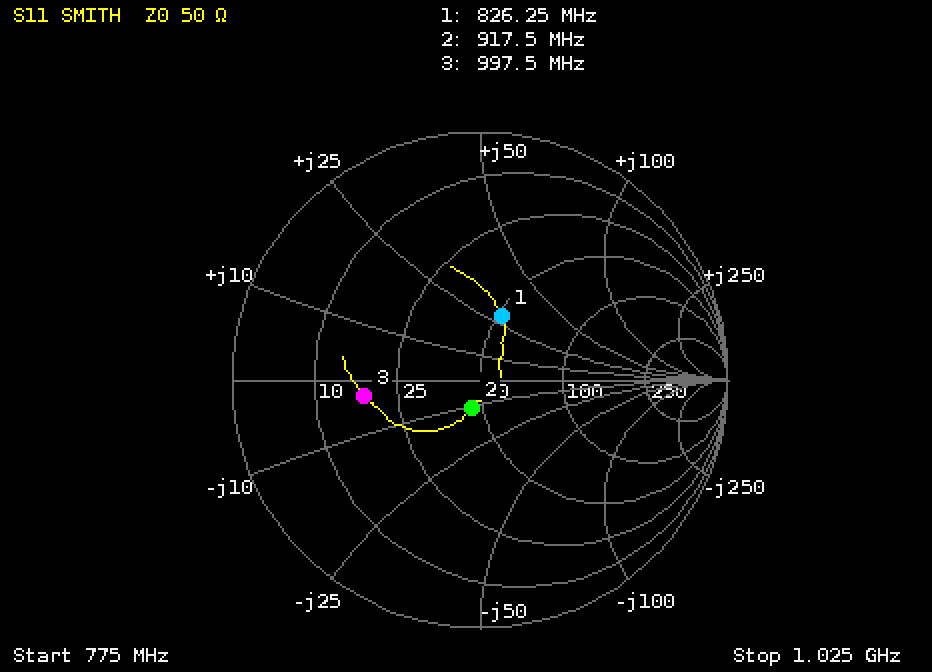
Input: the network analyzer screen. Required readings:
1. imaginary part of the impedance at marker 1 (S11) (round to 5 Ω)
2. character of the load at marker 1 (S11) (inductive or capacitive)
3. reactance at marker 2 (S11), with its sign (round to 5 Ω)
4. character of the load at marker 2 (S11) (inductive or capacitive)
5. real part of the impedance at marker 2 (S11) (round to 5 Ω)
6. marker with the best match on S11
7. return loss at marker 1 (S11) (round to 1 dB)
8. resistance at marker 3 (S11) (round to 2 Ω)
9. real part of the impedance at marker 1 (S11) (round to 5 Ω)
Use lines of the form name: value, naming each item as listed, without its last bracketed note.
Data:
imaginary part of the impedance at marker 1 (S11): +30 Ω
character of the load at marker 1 (S11): inductive
reactance at marker 2 (S11), with its sign: -10 Ω
character of the load at marker 2 (S11): capacitive
real part of the impedance at marker 2 (S11): 45 Ω
marker with the best match on S11: marker 2
return loss at marker 1 (S11): 11 dB
resistance at marker 3 (S11): 18 Ω
real part of the impedance at marker 1 (S11): 50 Ω
